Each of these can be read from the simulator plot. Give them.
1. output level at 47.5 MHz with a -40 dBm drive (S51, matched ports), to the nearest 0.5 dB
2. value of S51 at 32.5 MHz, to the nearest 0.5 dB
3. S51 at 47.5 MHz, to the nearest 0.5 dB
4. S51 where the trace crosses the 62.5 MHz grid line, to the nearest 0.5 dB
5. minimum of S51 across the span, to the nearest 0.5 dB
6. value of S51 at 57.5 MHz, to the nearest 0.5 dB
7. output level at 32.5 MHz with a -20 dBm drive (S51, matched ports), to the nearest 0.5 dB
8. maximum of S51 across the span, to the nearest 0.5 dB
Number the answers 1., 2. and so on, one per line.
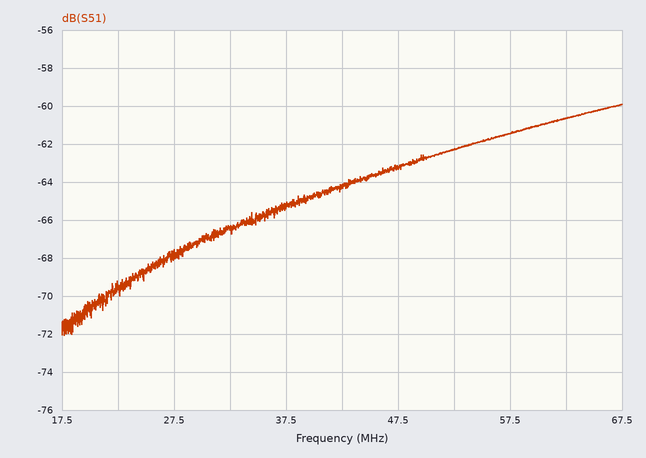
1. -103.0 dBm
2. -66.5 dB
3. -63.0 dB
4. -60.5 dB
5. -72.0 dB
6. -61.5 dB
7. -86.5 dBm
8. -60.0 dB
